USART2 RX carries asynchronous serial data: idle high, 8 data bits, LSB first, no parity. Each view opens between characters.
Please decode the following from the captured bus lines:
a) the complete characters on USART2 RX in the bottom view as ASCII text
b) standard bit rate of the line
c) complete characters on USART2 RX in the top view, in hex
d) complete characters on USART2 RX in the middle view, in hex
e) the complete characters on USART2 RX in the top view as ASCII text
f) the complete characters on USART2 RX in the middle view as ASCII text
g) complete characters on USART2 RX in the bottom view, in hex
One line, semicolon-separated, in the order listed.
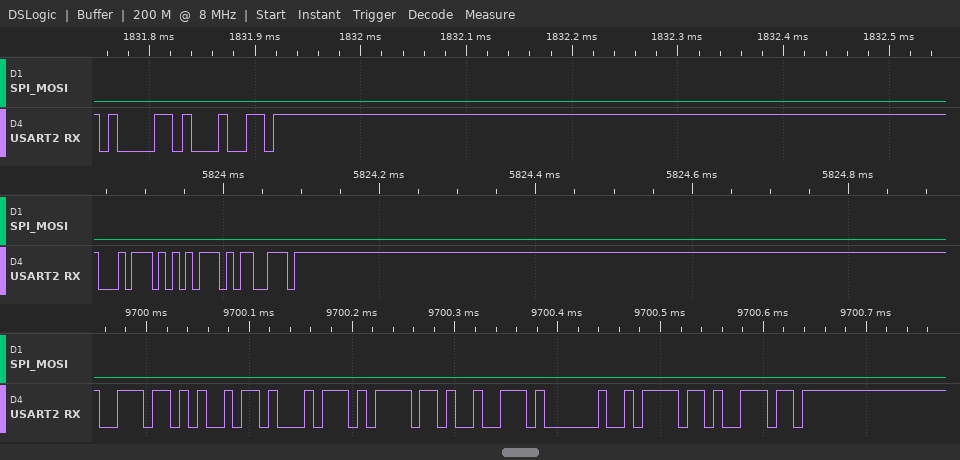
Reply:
"nitor on"; 115200 baud; 61, 64; 74, 75, 73; "ad"; "tus"; 6E, 69, 74, 6F, 72, 20, 6F, 6E
